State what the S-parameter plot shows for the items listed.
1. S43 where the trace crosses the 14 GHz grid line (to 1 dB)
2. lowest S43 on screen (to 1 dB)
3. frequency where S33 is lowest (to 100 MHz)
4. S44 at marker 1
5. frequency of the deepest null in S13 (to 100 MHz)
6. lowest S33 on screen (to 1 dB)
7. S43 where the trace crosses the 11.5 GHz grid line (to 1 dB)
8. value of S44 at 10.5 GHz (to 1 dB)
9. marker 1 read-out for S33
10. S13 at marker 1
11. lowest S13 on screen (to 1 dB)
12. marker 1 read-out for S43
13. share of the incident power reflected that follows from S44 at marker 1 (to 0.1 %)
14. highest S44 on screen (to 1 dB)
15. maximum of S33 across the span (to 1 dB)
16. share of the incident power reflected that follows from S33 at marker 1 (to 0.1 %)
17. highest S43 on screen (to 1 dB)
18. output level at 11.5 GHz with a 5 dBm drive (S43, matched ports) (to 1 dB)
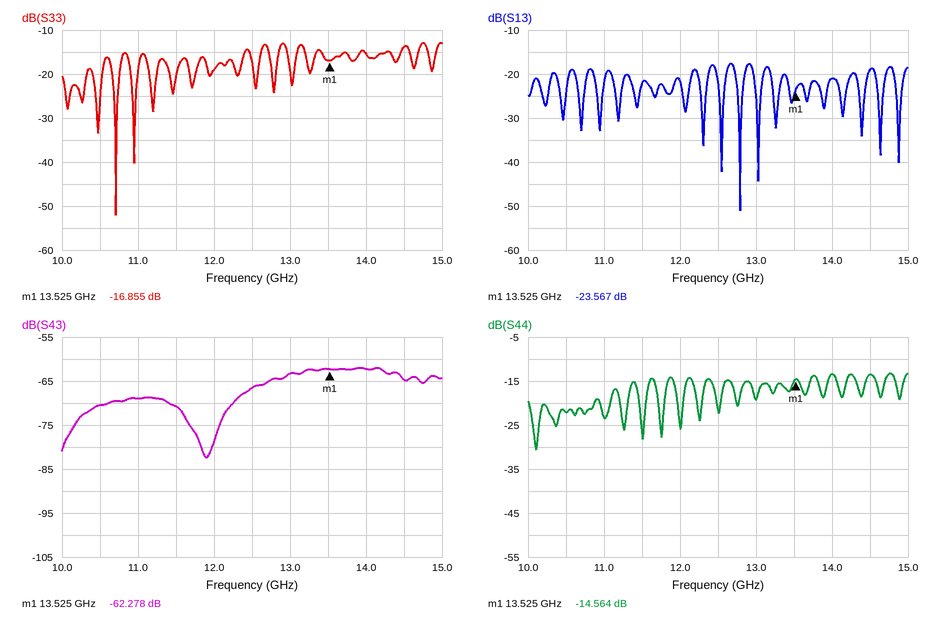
-62 dB
-82 dB
10.7 GHz
-14.564 dB
12.8 GHz
-52 dB
-71 dB
-22 dB
-16.855 dB
-23.567 dB
-51 dB
-62.278 dB
3.5 %
-13 dB
-13 dB
2.1 %
-62 dB
-66 dBm
